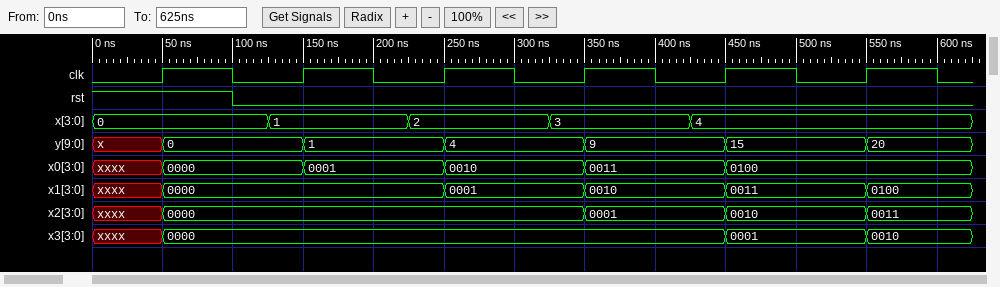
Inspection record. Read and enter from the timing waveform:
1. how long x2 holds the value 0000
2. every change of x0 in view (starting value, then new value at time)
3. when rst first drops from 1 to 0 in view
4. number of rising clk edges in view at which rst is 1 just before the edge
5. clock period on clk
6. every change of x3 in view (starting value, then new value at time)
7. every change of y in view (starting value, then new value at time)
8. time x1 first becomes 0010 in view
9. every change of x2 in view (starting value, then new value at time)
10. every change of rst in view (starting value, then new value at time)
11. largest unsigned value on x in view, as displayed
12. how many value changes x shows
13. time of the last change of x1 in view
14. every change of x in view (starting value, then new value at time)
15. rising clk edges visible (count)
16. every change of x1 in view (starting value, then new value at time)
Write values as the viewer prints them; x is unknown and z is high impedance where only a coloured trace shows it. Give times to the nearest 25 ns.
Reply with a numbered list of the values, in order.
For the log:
1. 300 ns
2. xxxx, 0000 at 50 ns, 0001 at 150 ns, 0010 at 250 ns, 0011 at 350 ns, 0100 at 450 ns
3. 100 ns
4. 1
5. 100 ns
6. xxxx, 0000 at 50 ns, 0001 at 450 ns, 0010 at 550 ns
7. x, 0 at 50 ns, 1 at 150 ns, 4 at 250 ns, 9 at 350 ns, 15 at 450 ns, 20 at 550 ns
8. 350 ns
9. xxxx, 0000 at 50 ns, 0001 at 350 ns, 0010 at 450 ns, 0011 at 550 ns
10. 1, 0 at 100 ns
11. 4
12. 4
13. 550 ns
14. 0, 1 at 125 ns, 2 at 225 ns, 3 at 325 ns, 4 at 425 ns
15. 6
16. xxxx, 0000 at 50 ns, 0001 at 250 ns, 0010 at 350 ns, 0011 at 450 ns, 0100 at 550 ns
